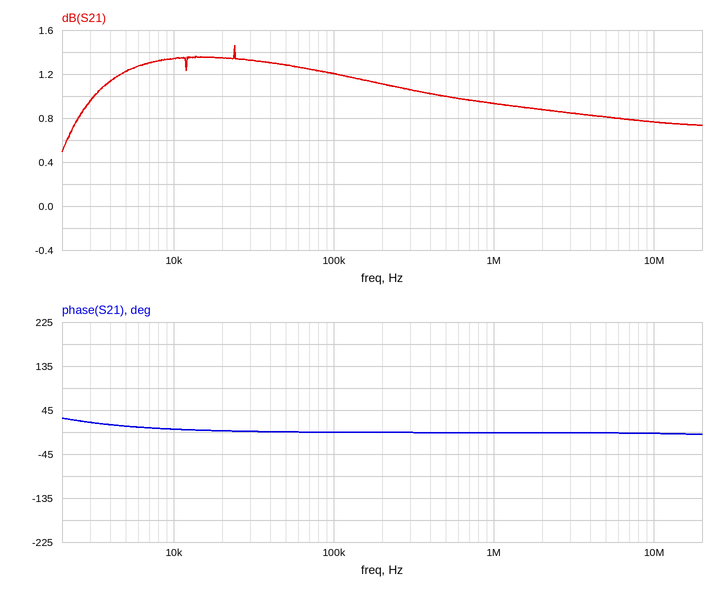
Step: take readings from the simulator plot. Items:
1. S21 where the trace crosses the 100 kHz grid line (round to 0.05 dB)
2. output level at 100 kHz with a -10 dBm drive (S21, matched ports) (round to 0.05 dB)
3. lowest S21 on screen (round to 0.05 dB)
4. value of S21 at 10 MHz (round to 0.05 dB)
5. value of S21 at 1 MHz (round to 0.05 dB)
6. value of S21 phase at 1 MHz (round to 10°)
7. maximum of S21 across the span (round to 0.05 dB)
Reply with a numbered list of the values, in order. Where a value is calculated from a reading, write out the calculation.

1. 1.20 dB
2. -10 dBm + (1.20 dB) = -8.80 dBm
3. 0.50 dB
4. 0.75 dB
5. 0.95 dB
6. 0°
7. 1.45 dB
